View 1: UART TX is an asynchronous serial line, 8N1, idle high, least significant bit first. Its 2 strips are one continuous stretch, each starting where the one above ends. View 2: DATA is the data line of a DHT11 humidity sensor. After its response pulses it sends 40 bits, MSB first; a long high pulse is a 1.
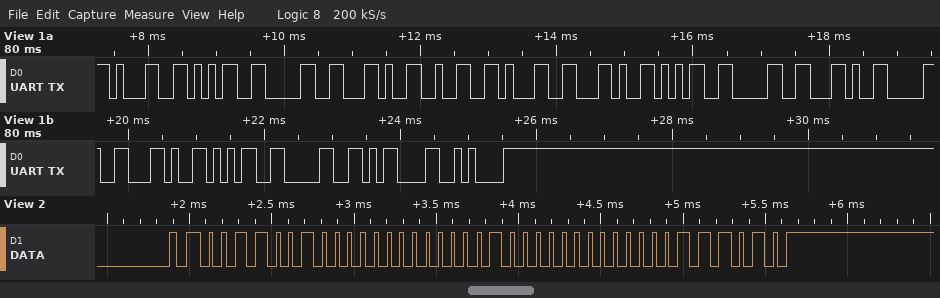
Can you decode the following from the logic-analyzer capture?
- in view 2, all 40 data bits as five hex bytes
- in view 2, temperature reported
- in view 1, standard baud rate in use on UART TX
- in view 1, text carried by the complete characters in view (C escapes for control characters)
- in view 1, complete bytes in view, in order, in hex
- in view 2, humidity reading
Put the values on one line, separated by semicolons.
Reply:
32 00 08 00 3A; 8.0 °C; 9600 baud; "150,21,50,0,50\r\n"; 31 35 30 2C 32 31 2C 35 30 2C 30 2C 35 30 0D 0A; 50 %
